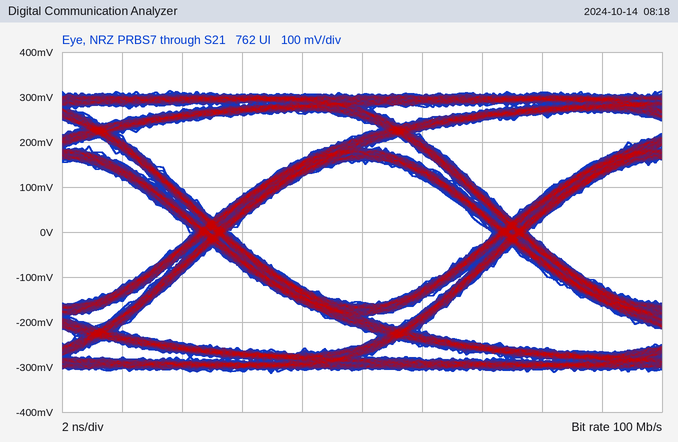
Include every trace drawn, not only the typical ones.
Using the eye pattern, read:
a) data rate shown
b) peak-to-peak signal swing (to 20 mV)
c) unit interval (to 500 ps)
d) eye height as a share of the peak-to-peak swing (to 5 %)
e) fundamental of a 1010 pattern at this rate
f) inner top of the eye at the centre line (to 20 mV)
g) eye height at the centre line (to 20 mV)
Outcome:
100 Mb/s
620 mV
10.0 ns
50 %
50 MHz
160 mV
320 mV
